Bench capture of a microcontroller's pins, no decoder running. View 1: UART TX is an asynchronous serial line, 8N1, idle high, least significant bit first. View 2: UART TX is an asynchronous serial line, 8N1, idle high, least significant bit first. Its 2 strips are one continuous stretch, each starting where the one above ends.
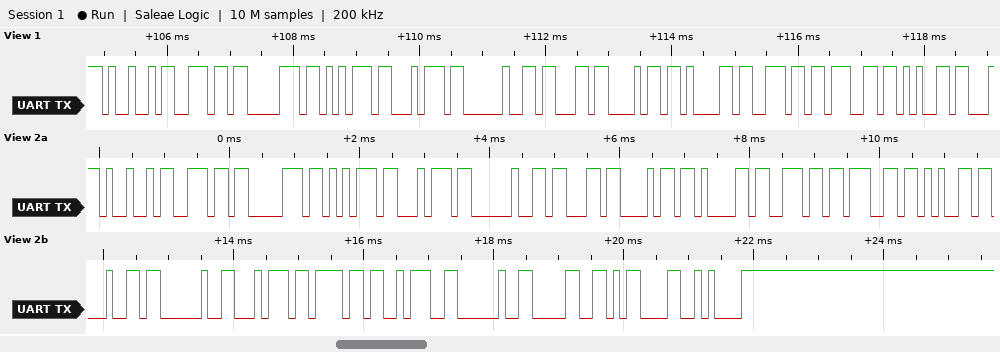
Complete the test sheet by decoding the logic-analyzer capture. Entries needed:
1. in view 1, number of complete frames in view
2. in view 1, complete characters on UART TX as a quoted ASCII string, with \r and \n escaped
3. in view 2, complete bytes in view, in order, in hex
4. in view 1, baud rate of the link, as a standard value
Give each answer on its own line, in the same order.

12
"Input change"
49 6E 70 75 74 20 63 68 61 6E 67 65 64 20 74 6F 3A 20 30 0D 0A
9600 baud
